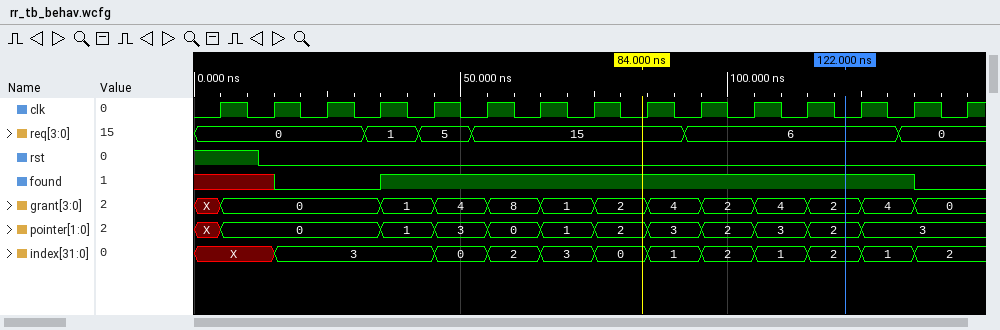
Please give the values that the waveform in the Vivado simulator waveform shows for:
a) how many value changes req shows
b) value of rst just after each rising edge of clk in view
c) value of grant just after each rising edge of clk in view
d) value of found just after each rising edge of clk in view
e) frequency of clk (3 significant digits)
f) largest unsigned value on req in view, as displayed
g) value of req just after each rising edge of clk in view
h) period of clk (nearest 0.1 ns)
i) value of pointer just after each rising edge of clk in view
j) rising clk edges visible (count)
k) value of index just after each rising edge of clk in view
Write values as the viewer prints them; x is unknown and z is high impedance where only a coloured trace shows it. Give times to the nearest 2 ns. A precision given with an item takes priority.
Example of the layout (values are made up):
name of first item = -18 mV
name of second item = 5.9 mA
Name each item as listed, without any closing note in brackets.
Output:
how many value changes req shows = 5
value of rst just after each rising edge of clk in view = 1 0 0 0 0 0 0 0 0 0 0 0 0 0 0
value of grant just after each rising edge of clk in view = 0, 0, 0, 1, 4, 8, 1, 2, 4, 2, 4, 2, 4, 0, 0
value of found just after each rising edge of clk in view = x 0 0 1 1 1 1 1 1 1 1 1 1 0 0
frequency of clk = 100 MHz
largest unsigned value on req in view, as displayed = 15
value of req just after each rising edge of clk in view = 0, 0, 0, 1, 5, 15, 15, 15, 15, 6, 6, 6, 6, 0, 0
period of clk = 10 ns
value of pointer just after each rising edge of clk in view = 0, 0, 0, 1, 3, 0, 1, 2, 3, 2, 3, 2, 3, 3, 3
rising clk edges visible = 15
value of index just after each rising edge of clk in view = X, 3, 3, 3, 0, 2, 3, 0, 1, 2, 1, 2, 1, 2, 2
